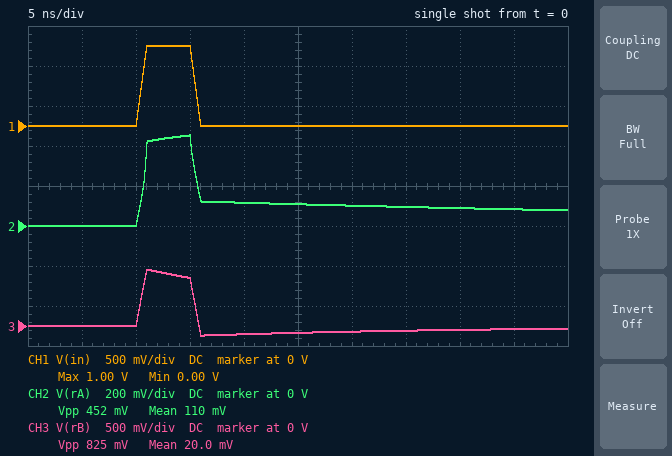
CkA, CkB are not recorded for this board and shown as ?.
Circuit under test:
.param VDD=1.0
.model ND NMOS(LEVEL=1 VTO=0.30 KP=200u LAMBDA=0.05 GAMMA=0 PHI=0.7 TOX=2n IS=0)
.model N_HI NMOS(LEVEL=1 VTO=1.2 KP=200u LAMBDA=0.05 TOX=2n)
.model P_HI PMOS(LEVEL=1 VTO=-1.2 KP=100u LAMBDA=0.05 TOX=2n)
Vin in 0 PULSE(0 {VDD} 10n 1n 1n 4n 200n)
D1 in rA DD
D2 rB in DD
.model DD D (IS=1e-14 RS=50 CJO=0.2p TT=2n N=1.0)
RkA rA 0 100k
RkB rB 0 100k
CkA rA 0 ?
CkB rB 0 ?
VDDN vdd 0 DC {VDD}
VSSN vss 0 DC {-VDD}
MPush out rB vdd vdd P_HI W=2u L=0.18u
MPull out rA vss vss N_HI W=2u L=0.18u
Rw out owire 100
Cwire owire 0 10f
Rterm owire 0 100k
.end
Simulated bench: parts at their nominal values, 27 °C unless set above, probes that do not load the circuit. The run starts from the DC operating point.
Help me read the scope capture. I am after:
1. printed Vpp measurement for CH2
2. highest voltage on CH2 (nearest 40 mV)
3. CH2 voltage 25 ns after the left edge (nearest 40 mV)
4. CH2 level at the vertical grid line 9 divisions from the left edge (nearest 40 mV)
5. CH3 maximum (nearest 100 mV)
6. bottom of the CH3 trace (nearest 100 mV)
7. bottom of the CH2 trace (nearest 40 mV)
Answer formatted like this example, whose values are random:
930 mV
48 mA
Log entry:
452 mV
440 mV
120 mV
80 mV
700 mV
-100 mV
0 V
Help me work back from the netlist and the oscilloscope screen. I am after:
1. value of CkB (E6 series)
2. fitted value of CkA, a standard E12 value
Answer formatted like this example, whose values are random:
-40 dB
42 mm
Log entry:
68 fF
560 fF
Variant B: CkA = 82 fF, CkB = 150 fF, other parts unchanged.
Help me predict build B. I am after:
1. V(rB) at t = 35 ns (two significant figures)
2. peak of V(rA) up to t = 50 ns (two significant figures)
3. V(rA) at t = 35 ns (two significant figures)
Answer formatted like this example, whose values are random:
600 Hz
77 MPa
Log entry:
-41 mV
700 mV
-58 mV
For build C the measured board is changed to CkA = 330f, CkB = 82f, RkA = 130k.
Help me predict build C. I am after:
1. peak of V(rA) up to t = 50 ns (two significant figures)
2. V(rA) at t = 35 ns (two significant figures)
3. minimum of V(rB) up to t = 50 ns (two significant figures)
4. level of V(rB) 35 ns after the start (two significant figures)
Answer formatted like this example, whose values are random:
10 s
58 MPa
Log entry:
470 mV
28 mV
-110 mV
-55 mV
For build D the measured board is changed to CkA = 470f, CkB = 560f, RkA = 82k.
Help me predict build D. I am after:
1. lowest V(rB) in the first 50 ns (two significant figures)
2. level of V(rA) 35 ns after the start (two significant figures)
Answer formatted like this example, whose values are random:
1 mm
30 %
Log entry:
-15 mV
63 mV
